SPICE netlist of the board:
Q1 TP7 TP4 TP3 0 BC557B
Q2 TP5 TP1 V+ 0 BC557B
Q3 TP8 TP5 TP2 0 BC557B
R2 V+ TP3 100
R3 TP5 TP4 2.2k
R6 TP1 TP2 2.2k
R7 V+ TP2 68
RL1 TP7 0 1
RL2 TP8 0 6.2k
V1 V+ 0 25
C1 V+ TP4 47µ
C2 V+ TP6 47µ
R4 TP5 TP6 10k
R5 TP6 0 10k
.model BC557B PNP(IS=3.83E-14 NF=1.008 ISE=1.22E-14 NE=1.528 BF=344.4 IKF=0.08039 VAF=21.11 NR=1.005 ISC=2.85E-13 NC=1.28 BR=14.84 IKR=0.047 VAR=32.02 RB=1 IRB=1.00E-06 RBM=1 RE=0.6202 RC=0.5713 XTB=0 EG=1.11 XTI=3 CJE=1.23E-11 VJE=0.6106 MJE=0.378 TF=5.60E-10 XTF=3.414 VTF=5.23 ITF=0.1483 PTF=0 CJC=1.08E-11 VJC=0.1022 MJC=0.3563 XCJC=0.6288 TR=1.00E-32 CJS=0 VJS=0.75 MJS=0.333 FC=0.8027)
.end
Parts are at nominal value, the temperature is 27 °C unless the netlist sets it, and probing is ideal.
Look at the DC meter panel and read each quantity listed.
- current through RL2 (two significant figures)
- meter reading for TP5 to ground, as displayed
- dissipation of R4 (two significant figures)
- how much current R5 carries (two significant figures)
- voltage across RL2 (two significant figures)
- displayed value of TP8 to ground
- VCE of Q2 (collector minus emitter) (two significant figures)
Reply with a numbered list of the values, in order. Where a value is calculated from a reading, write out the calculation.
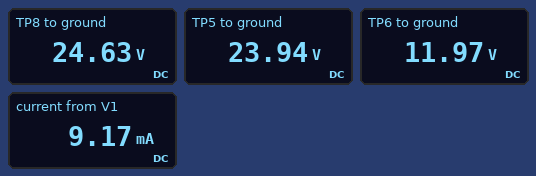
1. (24.63 V) / 6.2 kΩ = 4.0 mA
2. 23.94 V
3. (23.94 V - 11.97 V)^2 / 10 kΩ = 14 mW
4. (11.97 V) / 10 kΩ = 1.2 mA
5. 24.63 V = 25 V
6. 24.63 V
7. 23.94 V - 25 V = -1.1 V
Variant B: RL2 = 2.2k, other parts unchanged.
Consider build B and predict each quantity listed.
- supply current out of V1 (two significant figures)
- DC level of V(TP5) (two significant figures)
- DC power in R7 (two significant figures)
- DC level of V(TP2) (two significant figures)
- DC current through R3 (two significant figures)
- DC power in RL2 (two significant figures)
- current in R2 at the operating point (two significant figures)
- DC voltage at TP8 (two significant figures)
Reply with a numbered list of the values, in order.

1. 17 mA
2. 24 V
3. 6.0 mW
4. 24 V
5. 9.4 µA
6. 190 mW
7. 6.5 mA
8. 21 V
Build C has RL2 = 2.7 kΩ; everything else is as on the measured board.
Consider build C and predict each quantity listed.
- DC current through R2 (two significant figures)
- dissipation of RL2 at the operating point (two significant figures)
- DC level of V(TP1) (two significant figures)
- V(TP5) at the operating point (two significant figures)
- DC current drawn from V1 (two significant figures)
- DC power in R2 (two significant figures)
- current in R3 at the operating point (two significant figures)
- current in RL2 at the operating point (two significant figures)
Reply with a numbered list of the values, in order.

1. 6.5 mA
2. 220 mW
3. 24 V
4. 24 V
5. 17 mA
6. 4.2 mW
7. 9.5 µA
8. 9.0 mA
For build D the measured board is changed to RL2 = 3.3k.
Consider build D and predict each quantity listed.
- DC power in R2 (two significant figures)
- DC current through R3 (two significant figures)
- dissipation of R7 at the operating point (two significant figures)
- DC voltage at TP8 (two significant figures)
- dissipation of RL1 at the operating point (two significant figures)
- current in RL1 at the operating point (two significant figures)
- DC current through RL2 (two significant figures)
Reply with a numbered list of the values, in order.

1. 3.7 mW
2. 8.9 µA
3. 4.8 mW
4. 24 V
5. 37 µW
6. 6.1 mA
7. 7.4 mA
